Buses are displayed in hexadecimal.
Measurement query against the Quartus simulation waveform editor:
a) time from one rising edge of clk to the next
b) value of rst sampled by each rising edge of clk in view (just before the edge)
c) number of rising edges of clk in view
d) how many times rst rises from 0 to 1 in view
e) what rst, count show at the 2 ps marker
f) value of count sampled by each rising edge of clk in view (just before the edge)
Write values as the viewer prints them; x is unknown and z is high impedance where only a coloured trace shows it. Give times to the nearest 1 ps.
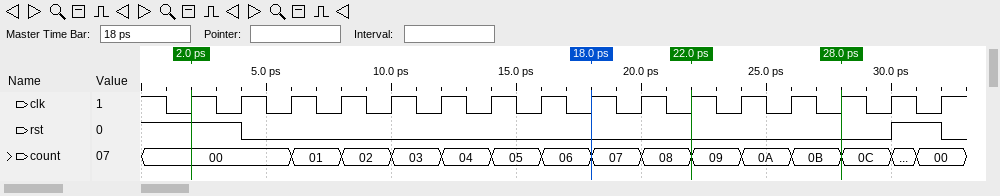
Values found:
2 ps
1 1 0 0 0 0 0 0 0 0 0 0 0 0 0 1
16
1
rst=1, count=00
00, 00, 00, 01, 02, 03, 04, 05, 06, 07, 08, 09, 0A, 0B, 0C, 00
